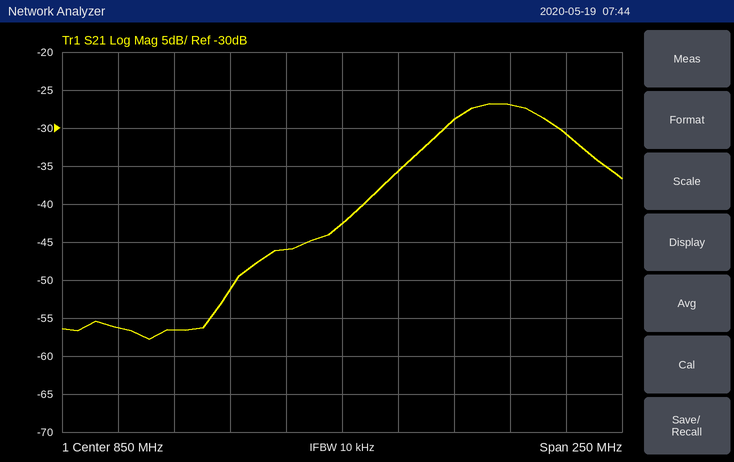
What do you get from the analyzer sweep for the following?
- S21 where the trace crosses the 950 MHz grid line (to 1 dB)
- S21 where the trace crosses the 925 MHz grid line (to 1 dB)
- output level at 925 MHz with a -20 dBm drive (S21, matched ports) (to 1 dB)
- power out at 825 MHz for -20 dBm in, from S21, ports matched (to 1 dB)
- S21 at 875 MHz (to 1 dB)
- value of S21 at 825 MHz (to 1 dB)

-31 dB
-27 dB
-47 dBm
-66 dBm
-36 dB
-46 dB
